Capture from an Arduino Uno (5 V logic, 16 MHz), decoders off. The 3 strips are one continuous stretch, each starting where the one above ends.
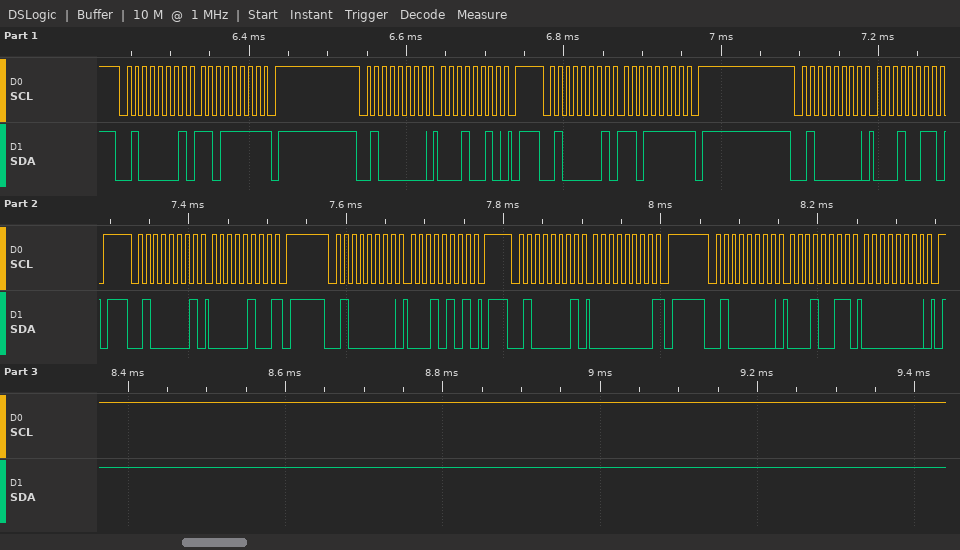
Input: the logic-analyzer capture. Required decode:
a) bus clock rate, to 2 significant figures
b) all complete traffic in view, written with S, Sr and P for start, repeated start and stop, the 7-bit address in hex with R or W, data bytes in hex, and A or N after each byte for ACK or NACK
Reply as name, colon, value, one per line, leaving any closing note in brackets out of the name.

bus clock rate, to 2 significant figures: 100 kHz
all complete traffic in view, written with S, Sr and P for start, repeated start and stop, the 7-bit address in hex with R or W, data bytes in hex, and A or N after each byte for ACK or NACK: S 20R A DF N P S 20W A 12 A P S 20R A DF N P S 20W A 13 A P S 20R A 04 N P S 20W A 15 A P S 20R A 00 N P S 20W A 13 A 00 A P
